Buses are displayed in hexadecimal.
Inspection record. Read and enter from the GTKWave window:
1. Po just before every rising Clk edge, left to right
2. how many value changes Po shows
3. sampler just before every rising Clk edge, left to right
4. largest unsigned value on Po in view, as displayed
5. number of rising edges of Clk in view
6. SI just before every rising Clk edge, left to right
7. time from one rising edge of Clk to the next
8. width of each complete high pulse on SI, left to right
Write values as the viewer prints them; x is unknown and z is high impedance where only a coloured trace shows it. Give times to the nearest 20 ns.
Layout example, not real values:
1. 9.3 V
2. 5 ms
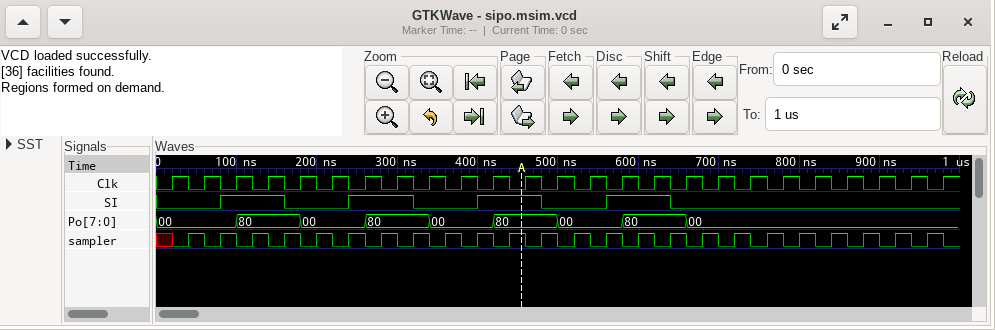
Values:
1. 00, 00, 00, 80, 80, 00, 00, 80, 80, 00, 00, 80, 80, 00, 00, 80, 80, 00, 00, 00, 00, 00, 00, 00, 00
2. 8
3. x 1 1 1 1 1 1 1 1 1 1 1 1 1 1 1 1 1 1 1 1 1 1 1 1
4. 80
5. 25
6. 0 0 1 1 0 0 1 1 0 0 1 1 0 0 1 1 0 0 0 0 0 0 0 0 0
7. 40 ns
8. 80 ns, 80 ns, 80 ns, 80 ns
